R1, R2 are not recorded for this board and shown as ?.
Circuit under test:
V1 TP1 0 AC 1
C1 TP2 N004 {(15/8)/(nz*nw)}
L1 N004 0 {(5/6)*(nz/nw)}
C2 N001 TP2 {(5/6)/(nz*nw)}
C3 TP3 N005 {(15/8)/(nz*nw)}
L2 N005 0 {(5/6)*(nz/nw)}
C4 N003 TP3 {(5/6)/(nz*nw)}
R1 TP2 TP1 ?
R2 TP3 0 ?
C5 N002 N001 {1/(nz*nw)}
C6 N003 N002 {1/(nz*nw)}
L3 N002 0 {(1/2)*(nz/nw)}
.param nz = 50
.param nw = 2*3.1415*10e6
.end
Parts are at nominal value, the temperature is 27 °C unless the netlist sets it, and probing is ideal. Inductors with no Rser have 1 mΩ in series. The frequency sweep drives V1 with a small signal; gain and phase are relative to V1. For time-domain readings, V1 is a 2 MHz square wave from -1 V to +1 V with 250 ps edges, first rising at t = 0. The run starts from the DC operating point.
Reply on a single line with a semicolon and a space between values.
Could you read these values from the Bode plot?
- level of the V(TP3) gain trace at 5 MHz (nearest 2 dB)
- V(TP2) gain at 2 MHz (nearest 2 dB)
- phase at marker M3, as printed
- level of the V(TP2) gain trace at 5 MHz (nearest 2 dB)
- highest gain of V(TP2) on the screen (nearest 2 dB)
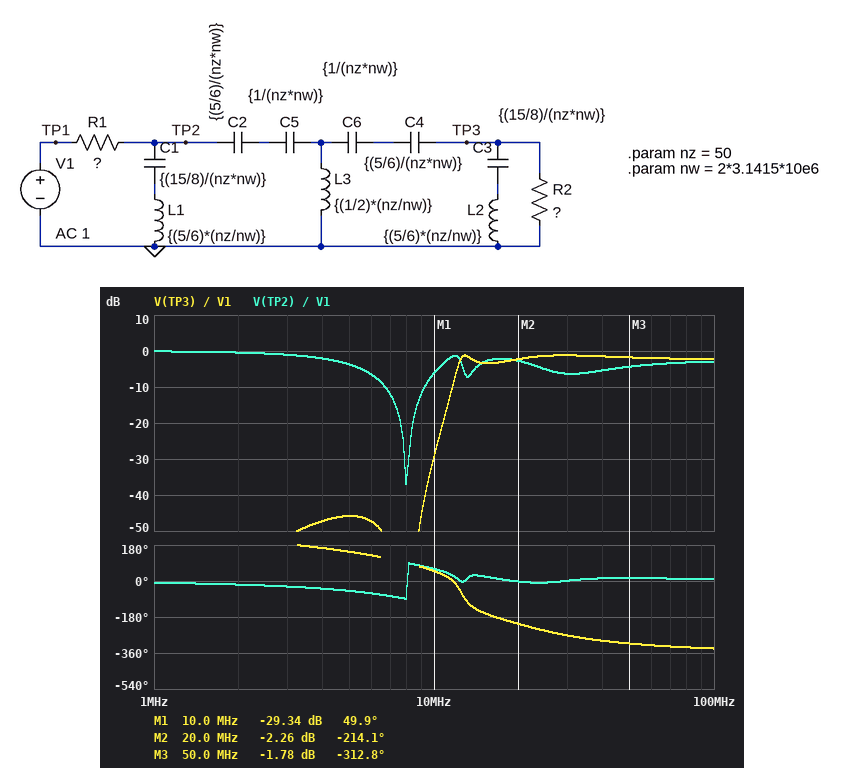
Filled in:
-46 dB; 0 dB; -312.8 deg; -4 dB; 0 dB
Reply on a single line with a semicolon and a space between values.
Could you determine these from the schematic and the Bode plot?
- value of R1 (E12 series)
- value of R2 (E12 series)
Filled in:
33 Ω; 100 Ω
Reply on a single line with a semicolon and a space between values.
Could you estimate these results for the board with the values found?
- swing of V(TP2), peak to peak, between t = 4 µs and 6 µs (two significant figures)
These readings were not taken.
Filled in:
2.3 V
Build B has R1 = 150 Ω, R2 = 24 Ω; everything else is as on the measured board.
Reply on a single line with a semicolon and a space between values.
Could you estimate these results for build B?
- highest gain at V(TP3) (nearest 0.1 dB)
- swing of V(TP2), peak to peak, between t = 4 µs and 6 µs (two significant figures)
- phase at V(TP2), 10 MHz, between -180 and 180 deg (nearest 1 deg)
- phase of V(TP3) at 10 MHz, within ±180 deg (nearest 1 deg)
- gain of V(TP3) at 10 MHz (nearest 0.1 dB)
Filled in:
-14.0 dB; 1.7 V; 83 deg; 45 deg; -43.3 dB
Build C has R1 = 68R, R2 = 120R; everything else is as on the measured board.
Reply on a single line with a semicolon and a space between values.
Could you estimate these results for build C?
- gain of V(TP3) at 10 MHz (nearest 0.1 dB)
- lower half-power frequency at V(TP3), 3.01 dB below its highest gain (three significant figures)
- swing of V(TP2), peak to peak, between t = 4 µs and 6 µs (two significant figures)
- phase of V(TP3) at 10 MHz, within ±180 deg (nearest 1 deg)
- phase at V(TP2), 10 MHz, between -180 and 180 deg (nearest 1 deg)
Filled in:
-34.7 dB; 12.0 MHz; 2.0 V; 66 deg; 75 deg
